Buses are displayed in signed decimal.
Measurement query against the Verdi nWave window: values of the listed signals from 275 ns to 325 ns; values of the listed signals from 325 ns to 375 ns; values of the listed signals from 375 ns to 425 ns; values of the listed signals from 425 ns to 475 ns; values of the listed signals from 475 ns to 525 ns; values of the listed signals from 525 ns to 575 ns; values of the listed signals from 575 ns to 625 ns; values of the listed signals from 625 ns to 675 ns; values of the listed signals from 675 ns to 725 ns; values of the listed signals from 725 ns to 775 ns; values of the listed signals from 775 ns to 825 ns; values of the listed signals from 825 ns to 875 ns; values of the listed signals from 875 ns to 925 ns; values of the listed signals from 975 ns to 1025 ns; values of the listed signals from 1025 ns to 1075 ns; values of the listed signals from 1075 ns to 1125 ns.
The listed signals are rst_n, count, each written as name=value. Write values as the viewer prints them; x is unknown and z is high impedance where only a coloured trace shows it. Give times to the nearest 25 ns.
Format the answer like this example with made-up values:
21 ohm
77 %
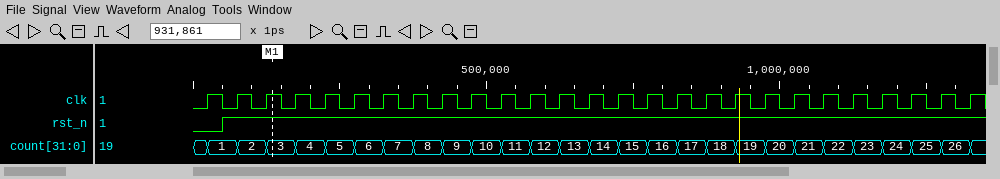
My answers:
rst_n=1, count=6
rst_n=1, count=7
rst_n=1, count=8
rst_n=1, count=9
rst_n=1, count=10
rst_n=1, count=11
rst_n=1, count=12
rst_n=1, count=13
rst_n=1, count=14
rst_n=1, count=15
rst_n=1, count=16
rst_n=1, count=17
rst_n=1, count=18
rst_n=1, count=20
rst_n=1, count=21
rst_n=1, count=22
